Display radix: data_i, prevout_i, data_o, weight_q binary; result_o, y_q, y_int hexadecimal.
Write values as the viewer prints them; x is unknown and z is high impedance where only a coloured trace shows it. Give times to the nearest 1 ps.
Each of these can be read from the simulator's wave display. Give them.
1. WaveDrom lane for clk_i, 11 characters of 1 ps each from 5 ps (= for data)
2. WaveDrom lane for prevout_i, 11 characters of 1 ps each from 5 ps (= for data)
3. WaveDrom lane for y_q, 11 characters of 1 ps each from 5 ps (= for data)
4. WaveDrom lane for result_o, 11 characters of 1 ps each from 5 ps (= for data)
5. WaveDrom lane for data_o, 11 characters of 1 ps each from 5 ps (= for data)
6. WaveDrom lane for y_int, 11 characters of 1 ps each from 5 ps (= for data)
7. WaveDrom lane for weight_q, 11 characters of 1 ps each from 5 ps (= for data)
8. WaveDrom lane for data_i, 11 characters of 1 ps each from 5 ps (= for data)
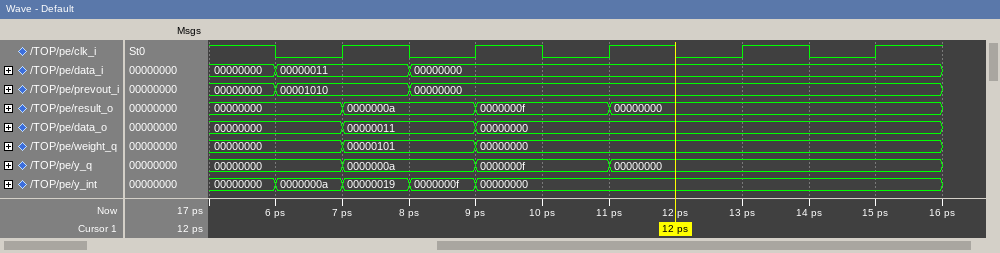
{name: 'clk_i', wave: '10101010101'}
{name: 'prevout_i', wave: '==.=.......', data: '00000000 00001010 00000000'}
{name: 'y_q', wave: '=.=.=.=....', data: '00000000 0000000a 0000000f 00000000'}
{name: 'result_o', wave: '=.=.=.=....', data: '00000000 0000000a 0000000f 00000000'}
{name: 'data_o', wave: '=.=.=......', data: '00000000 00000011 00000000'}
{name: 'y_int', wave: '=====......', data: '00000000 0000000a 00000019 0000000f 00000000'}
{name: 'weight_q', wave: '=.=.=......', data: '00000000 00000101 00000000'}
{name: 'data_i', wave: '==.=.......', data: '00000000 00000011 00000000'}
